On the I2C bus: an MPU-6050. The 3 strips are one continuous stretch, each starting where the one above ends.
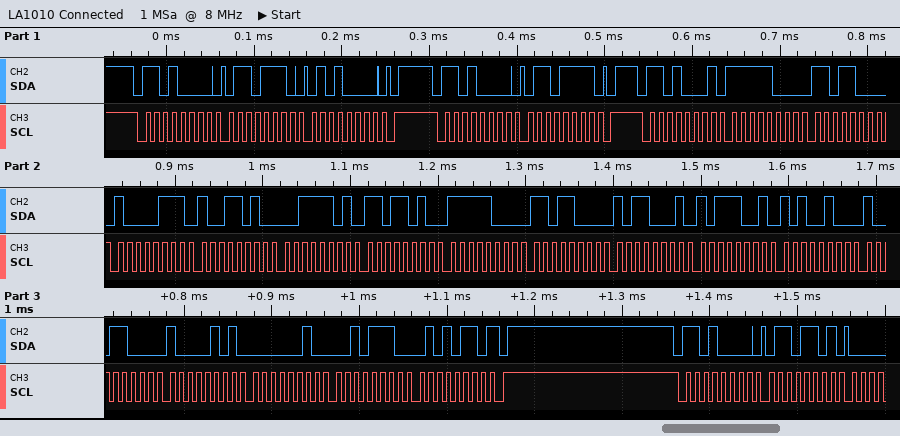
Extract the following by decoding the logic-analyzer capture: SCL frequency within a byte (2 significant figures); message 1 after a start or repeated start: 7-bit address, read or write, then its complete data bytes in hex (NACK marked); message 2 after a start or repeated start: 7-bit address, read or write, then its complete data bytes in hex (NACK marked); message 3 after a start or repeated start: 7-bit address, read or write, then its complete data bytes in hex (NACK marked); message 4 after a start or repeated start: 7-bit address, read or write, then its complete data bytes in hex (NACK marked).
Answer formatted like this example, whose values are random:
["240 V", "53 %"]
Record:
["100 kHz", "0x68 write: 6E 50", "0x68 write: 6F", "0x68 read: F8 D8 87 9A 3D DA F8 D8 B1 B9 A4 98 85 02 2E 56 NACK", "0x68 write: 6D"]
